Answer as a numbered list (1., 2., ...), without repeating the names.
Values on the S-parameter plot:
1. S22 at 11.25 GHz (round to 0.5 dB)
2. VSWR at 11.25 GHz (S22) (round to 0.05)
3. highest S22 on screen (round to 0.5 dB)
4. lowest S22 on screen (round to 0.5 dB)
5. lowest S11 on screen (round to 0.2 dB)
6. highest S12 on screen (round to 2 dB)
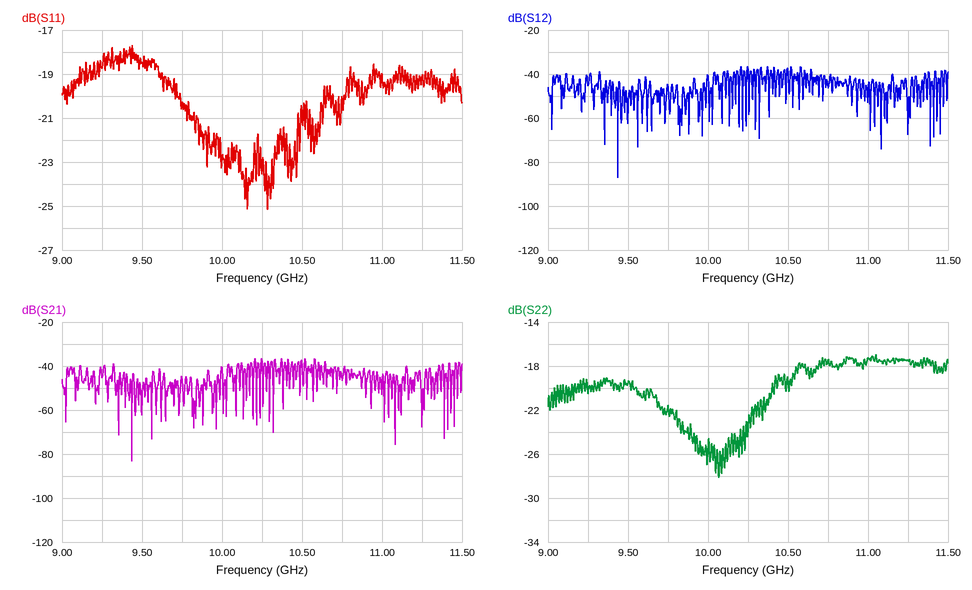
1. -17.5 dB
2. 1.30
3. -17.0 dB
4. -28.0 dB
5. -25.2 dB
6. -36 dB
